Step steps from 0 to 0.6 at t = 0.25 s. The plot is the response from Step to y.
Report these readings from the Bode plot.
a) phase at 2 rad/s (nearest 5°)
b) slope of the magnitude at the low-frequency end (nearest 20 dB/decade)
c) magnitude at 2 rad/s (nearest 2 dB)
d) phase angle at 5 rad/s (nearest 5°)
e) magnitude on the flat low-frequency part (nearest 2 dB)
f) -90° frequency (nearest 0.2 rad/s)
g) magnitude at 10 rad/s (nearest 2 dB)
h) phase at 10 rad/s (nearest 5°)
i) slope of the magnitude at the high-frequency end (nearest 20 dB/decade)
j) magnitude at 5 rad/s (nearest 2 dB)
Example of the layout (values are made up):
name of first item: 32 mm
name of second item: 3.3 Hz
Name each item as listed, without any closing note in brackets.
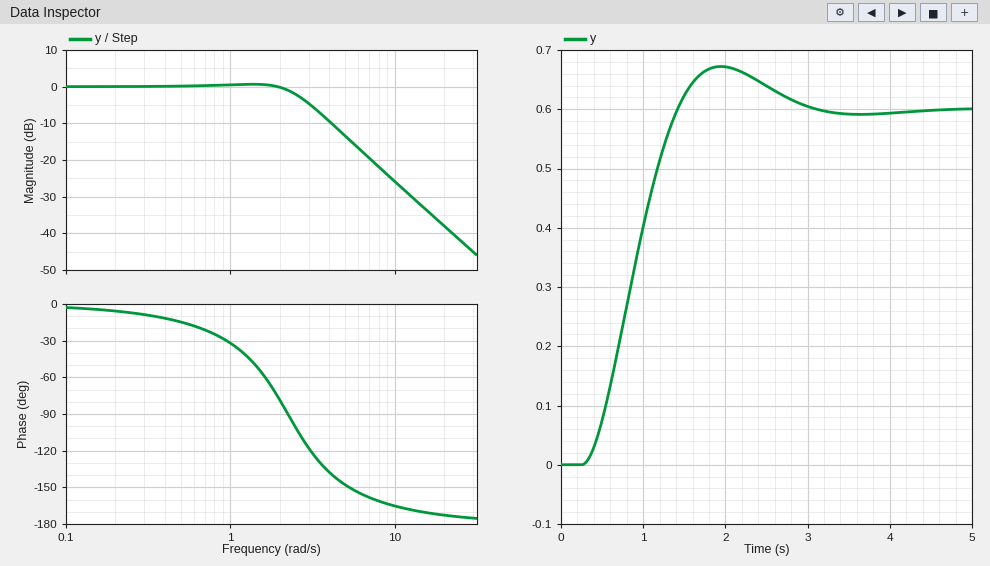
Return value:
phase at 2 rad/s: -80°
slope of the magnitude at the low-frequency end: 0 dB/decade
magnitude at 2 rad/s: 0 dB
phase angle at 5 rad/s: -150°
magnitude on the flat low-frequency part: 0 dB
-90° frequency: 2.2 rad/s
magnitude at 10 rad/s: -26 dB
phase at 10 rad/s: -165°
slope of the magnitude at the high-frequency end: -40 dB/decade
magnitude at 5 rad/s: -14 dB
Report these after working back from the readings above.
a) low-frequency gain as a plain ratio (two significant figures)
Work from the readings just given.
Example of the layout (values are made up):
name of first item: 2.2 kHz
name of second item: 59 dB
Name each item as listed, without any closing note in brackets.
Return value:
low-frequency gain as a plain ratio: 1.0
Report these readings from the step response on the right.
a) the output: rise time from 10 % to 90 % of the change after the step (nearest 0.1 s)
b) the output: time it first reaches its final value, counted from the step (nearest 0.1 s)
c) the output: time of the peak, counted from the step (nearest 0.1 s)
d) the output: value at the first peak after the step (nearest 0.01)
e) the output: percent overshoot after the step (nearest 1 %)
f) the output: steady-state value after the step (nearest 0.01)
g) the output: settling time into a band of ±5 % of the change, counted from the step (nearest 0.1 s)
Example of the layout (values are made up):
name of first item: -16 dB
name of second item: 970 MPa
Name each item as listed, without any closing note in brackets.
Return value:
the output: rise time from 10 % to 90 % of the change after the step: 0.8 s
the output: time it first reaches its final value, counted from the step: 1.2 s
the output: time of the peak, counted from the step: 1.7 s
the output: value at the first peak after the step: 0.67
the output: percent overshoot after the step: 12 %
the output: steady-state value after the step: 0.60
the output: settling time into a band of ±5 % of the change, counted from the step: 2.4 s
